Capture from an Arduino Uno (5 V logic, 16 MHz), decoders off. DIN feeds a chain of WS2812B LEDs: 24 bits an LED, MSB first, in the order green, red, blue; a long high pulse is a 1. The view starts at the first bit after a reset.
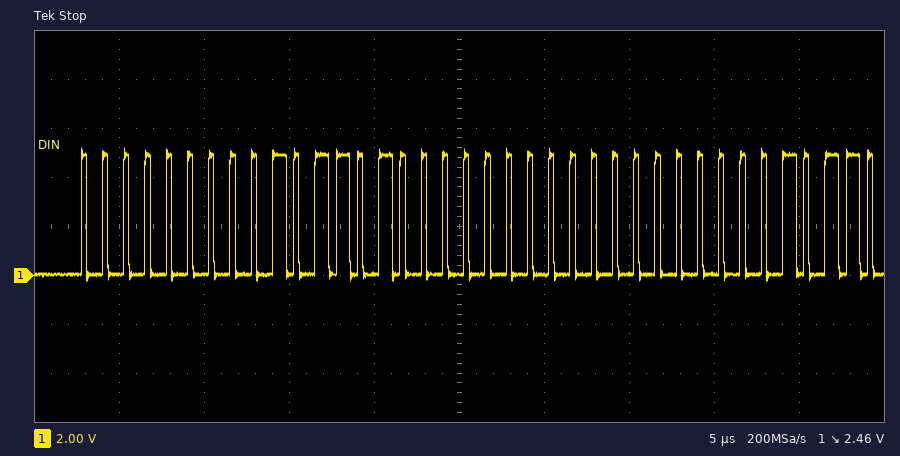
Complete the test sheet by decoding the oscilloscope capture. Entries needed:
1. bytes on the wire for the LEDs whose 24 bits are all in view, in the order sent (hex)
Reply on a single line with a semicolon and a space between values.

00 5A 00
